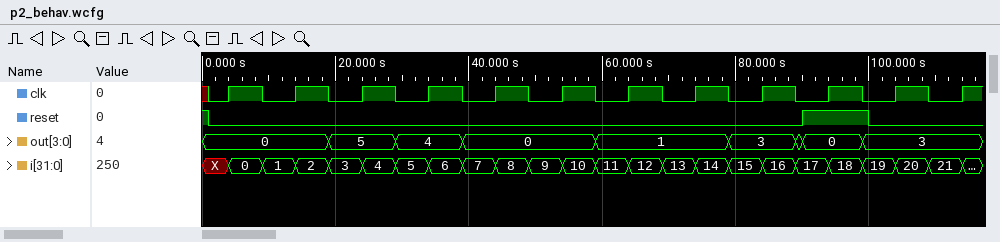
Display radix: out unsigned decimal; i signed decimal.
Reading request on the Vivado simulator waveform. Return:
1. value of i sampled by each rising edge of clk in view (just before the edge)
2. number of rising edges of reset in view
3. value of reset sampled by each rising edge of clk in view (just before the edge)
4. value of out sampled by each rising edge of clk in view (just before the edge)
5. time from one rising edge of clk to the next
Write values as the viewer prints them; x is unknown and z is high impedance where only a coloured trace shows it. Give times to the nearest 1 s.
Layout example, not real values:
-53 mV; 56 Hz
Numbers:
X, 1, 3, 5, 7, 9, 11, 13, 15, 17, 19, 21; 1; 0 0 0 0 0 0 0 0 0 1 0 0; 0, 0, 5, 4, 0, 0, 1, 1, 3, 0, 3, 3; 10 s
